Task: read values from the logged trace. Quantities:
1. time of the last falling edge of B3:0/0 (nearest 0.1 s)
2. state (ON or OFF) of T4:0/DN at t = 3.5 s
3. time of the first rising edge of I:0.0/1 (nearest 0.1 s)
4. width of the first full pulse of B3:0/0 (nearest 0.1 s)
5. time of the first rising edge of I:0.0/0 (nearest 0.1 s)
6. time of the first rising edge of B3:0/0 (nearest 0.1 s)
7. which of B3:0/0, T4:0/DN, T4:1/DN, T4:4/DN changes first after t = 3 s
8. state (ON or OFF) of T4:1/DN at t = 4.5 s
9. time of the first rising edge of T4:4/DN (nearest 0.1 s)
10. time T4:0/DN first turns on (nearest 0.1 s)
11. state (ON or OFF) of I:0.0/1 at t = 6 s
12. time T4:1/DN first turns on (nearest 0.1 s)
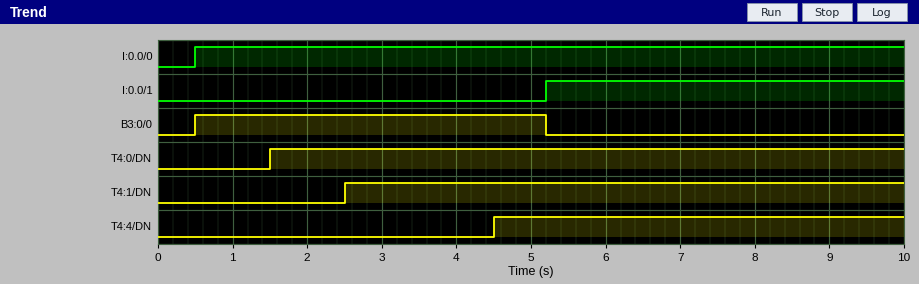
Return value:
5.2 s
ON
5.2 s
4.7 s
0.5 s
0.5 s
T4:4/DN
ON
4.5 s
1.5 s
ON
2.5 s
